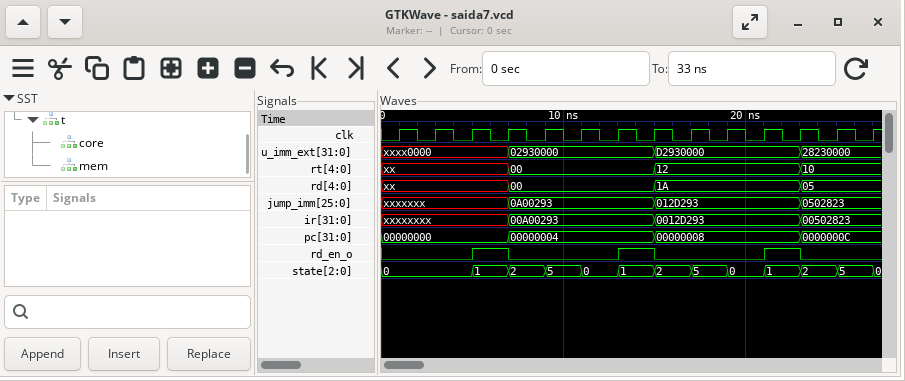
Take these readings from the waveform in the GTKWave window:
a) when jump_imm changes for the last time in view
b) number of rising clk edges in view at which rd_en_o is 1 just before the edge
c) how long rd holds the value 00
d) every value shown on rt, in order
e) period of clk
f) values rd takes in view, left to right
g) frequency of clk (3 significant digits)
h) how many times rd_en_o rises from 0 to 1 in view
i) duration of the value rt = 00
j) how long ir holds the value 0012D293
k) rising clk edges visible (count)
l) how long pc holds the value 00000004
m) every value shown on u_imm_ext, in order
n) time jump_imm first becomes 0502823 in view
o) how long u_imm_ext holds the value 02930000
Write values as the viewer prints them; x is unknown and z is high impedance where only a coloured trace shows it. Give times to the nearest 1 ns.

23 ns
3
8 ns
xx, 00, 12, 10
2 ns
xx, 00, 1A, 05
500 MHz
3
8 ns
8 ns
14
8 ns
xxxx0000, 02930000, D2930000, 28230000
23 ns
8 ns
